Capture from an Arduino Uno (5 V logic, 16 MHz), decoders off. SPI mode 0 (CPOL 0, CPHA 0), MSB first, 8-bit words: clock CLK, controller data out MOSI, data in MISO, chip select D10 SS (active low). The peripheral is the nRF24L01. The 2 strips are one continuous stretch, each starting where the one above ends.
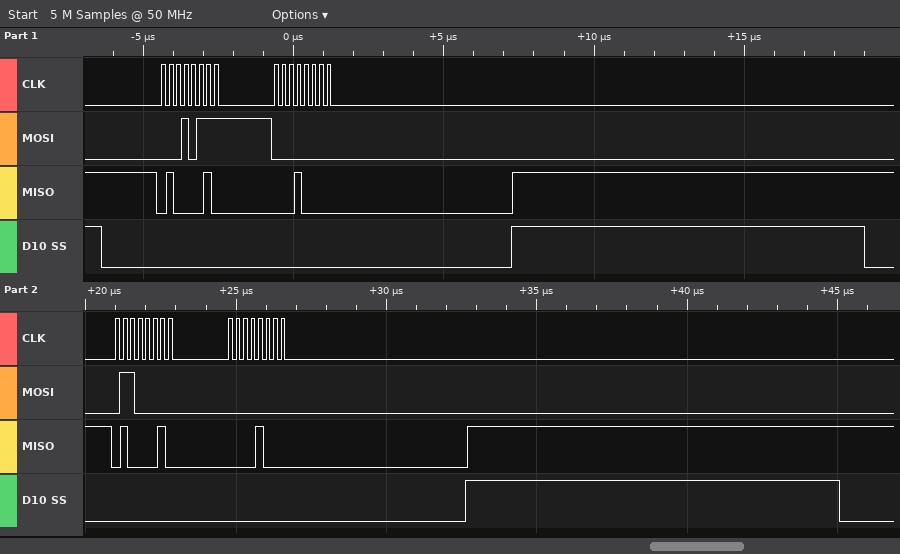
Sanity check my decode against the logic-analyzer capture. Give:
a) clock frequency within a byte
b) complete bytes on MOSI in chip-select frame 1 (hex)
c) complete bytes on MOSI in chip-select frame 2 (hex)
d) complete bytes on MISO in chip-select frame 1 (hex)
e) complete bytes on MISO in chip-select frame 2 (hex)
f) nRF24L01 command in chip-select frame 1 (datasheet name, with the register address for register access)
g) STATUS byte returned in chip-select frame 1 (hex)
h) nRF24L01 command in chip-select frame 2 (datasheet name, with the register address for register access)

4 MHz
17 00
60 00
42 10
42 08
R_REGISTER 0x17
0x42
R_RX_PL_WID
